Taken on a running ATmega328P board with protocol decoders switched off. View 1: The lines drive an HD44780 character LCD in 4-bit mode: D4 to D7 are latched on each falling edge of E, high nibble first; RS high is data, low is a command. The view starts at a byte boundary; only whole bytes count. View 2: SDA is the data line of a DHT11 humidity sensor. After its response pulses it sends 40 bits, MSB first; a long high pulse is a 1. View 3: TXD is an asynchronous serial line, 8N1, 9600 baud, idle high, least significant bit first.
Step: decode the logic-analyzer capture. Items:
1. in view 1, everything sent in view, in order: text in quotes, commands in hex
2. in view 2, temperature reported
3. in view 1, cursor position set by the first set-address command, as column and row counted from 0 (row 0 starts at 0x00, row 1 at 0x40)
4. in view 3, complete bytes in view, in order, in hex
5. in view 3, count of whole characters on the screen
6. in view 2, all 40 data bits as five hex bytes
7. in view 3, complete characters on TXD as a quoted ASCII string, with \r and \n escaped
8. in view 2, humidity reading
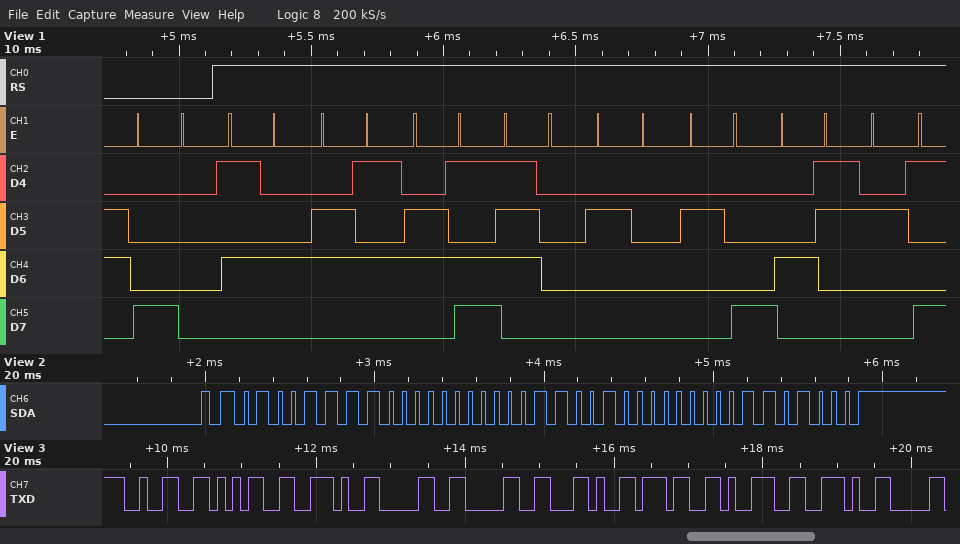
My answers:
0x80 "Temp (C)"
25.0 °C
column 0, row 0
32 35 2E 30 30 2C 37 39 2E
9
4F 00 19 00 68
"25.00,79."
79 %
